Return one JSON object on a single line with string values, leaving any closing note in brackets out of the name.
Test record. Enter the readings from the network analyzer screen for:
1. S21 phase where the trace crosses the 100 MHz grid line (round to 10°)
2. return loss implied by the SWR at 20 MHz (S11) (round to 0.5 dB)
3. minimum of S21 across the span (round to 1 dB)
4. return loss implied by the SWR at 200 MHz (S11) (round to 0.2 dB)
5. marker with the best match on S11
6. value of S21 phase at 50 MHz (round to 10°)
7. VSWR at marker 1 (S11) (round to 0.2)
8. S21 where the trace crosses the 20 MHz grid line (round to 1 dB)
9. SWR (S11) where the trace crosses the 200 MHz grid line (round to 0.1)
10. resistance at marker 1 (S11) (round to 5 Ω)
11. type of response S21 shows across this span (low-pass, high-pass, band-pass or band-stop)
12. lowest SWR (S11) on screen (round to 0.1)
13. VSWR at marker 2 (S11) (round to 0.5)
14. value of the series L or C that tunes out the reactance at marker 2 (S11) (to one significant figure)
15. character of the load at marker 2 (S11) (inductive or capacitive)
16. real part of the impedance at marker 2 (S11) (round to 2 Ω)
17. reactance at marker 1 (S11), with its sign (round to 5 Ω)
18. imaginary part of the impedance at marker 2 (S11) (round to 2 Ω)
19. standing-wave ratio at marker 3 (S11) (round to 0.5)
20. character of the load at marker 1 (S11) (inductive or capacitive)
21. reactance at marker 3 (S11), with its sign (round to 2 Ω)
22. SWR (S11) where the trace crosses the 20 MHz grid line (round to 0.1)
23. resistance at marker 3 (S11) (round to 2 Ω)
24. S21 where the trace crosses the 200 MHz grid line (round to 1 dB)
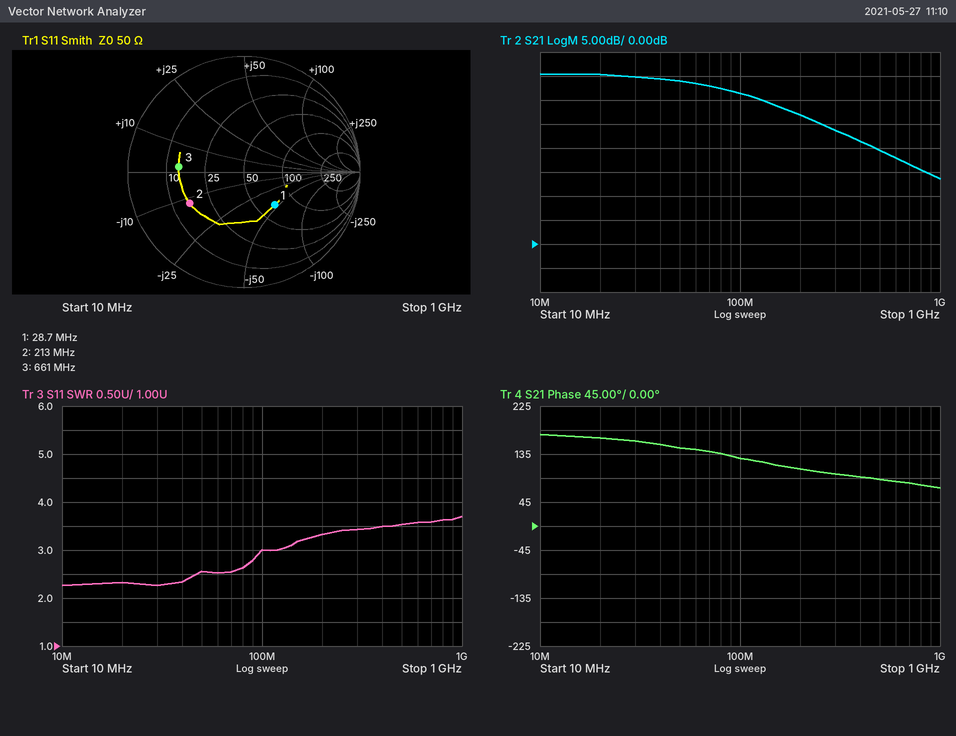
{"S21 phase where the trace crosses the 100 MHz grid line": "130°", "return loss implied by the SWR at 20 MHz (S11)": "8.0 dB", "minimum of S21 across the span": "14 dB", "return loss implied by the SWR at 200 MHz (S11)": "5.4 dB", "marker with the best match on S11": "marker 1", "value of S21 phase at 50 MHz": "150°", "VSWR at marker 1 (S11)": "2.2", "S21 where the trace crosses the 20 MHz grid line": "35 dB", "SWR (S11) where the trace crosses the 200 MHz grid line": "3.3", "resistance at marker 1 (S11)": "70 Ω", "type of response S21 shows across this span": "low-pass", "lowest SWR (S11) on screen": "2.3", "VSWR at marker 2 (S11)": "3.5", "value of the series L or C that tunes out the reactance at marker 2 (S11)": "9 nH", "character of the load at marker 2 (S11)": "capacitive", "real part of the impedance at marker 2 (S11)": "16 Ω", "reactance at marker 1 (S11), with its sign": "-45 Ω", "imaginary part of the impedance at marker 2 (S11)": "-12 Ω", "standing-wave ratio at marker 3 (S11)": "3.5", "character of the load at marker 1 (S11)": "capacitive", "reactance at marker 3 (S11), with its sign": "+2 Ω", "SWR (S11) where the trace crosses the 20 MHz grid line": "2.3", "resistance at marker 3 (S11)": "14 Ω", "S21 where the trace crosses the 200 MHz grid line": "27 dB"}
